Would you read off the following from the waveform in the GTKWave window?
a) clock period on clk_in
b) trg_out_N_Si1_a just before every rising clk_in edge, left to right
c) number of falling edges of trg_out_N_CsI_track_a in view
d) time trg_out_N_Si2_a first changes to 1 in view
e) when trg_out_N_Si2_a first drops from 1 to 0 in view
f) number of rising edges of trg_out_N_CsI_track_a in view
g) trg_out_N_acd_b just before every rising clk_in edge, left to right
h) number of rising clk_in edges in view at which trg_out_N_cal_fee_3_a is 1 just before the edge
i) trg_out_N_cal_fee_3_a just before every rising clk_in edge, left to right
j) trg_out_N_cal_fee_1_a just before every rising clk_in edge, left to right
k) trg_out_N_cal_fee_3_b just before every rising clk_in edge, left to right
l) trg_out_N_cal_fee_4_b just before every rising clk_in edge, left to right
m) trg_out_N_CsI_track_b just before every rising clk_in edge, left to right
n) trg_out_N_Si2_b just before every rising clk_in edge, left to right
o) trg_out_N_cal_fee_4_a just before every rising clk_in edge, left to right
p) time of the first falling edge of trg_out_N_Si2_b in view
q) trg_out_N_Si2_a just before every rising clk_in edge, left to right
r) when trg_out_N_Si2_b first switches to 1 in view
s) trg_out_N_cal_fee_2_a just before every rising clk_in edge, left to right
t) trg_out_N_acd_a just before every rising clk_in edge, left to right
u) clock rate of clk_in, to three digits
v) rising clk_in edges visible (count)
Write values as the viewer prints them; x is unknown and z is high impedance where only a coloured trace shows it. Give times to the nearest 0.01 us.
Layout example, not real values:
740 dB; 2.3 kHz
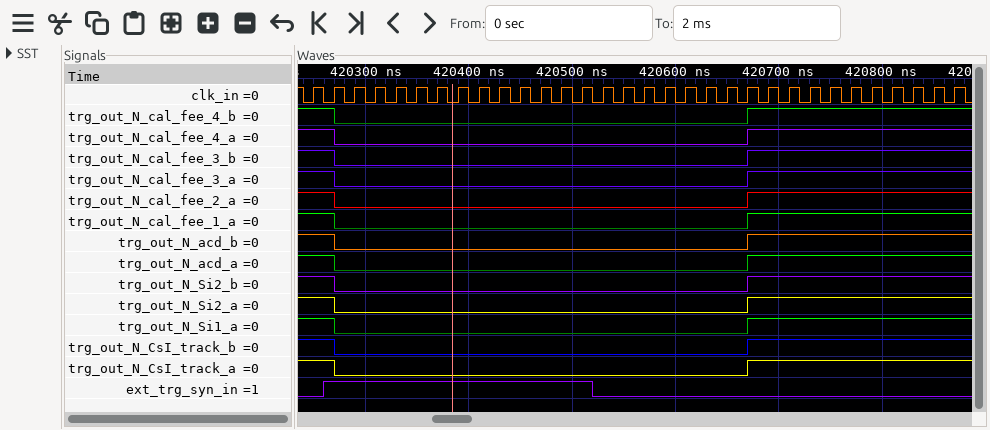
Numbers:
0.02 us; 1 1 0 0 0 0 0 0 0 0 0 0 0 0 0 0 0 0 0 0 0 0 1 1 1 1 1 1 1 1 1 1; 1; 420.67 us; 420.27 us; 1; 1 1 0 0 0 0 0 0 0 0 0 0 0 0 0 0 0 0 0 0 0 0 1 1 1 1 1 1 1 1 1 1; 12; 1 1 0 0 0 0 0 0 0 0 0 0 0 0 0 0 0 0 0 0 0 0 1 1 1 1 1 1 1 1 1 1; 1 1 0 0 0 0 0 0 0 0 0 0 0 0 0 0 0 0 0 0 0 0 1 1 1 1 1 1 1 1 1 1; 1 1 0 0 0 0 0 0 0 0 0 0 0 0 0 0 0 0 0 0 0 0 1 1 1 1 1 1 1 1 1 1; 1 1 0 0 0 0 0 0 0 0 0 0 0 0 0 0 0 0 0 0 0 0 1 1 1 1 1 1 1 1 1 1; 1 1 0 0 0 0 0 0 0 0 0 0 0 0 0 0 0 0 0 0 0 0 1 1 1 1 1 1 1 1 1 1; 1 1 0 0 0 0 0 0 0 0 0 0 0 0 0 0 0 0 0 0 0 0 1 1 1 1 1 1 1 1 1 1; 1 1 0 0 0 0 0 0 0 0 0 0 0 0 0 0 0 0 0 0 0 0 1 1 1 1 1 1 1 1 1 1; 420.27 us; 1 1 0 0 0 0 0 0 0 0 0 0 0 0 0 0 0 0 0 0 0 0 1 1 1 1 1 1 1 1 1 1; 420.67 us; 1 1 0 0 0 0 0 0 0 0 0 0 0 0 0 0 0 0 0 0 0 0 1 1 1 1 1 1 1 1 1 1; 1 1 0 0 0 0 0 0 0 0 0 0 0 0 0 0 0 0 0 0 0 0 1 1 1 1 1 1 1 1 1 1; 50.0 MHz; 32
